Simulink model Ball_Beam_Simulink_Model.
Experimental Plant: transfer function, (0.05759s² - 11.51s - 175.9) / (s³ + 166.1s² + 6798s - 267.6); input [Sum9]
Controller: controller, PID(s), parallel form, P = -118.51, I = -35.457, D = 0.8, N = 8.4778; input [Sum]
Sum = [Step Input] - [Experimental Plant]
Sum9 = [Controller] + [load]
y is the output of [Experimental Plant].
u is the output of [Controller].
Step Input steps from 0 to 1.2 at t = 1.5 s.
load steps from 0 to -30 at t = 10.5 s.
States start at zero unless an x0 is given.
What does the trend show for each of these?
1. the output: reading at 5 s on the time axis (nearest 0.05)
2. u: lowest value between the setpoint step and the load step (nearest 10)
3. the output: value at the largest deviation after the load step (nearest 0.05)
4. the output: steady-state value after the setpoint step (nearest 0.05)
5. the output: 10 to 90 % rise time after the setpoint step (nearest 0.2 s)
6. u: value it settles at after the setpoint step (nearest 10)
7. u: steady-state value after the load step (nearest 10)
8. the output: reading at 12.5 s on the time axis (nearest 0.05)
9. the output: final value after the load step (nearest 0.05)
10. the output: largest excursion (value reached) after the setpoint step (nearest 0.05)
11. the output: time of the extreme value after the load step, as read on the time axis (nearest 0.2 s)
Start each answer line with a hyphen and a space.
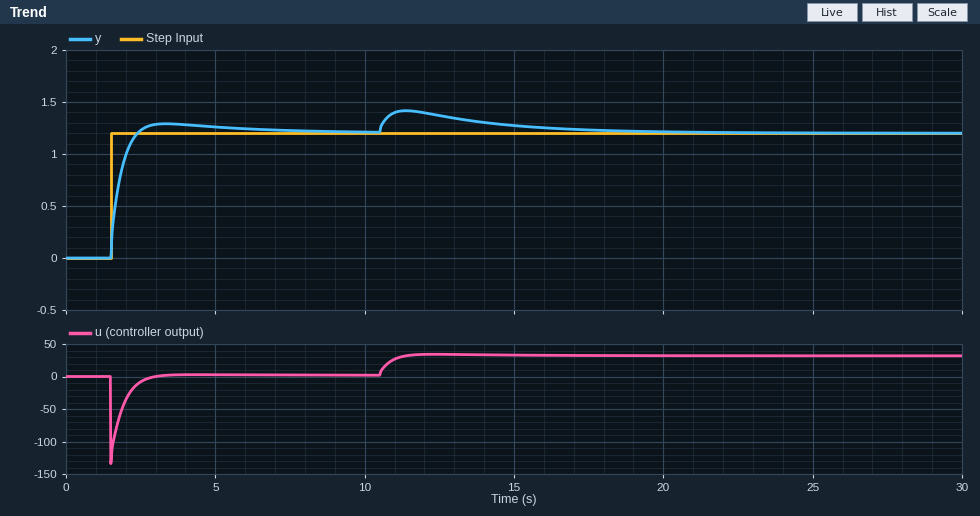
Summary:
- 1.25
- -130
- 1.40
- 1.20
- 0.6 s
- 0
- 30
- 1.35
- 1.20
- 1.30
- 11.4 s
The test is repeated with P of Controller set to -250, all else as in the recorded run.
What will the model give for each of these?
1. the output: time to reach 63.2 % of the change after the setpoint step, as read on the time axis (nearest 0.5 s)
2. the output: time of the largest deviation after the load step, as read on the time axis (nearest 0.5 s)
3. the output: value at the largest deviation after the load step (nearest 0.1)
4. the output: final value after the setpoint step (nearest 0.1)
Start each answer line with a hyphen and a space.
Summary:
- 1.5 s
- 11.0 s
- 1.3
- 1.2
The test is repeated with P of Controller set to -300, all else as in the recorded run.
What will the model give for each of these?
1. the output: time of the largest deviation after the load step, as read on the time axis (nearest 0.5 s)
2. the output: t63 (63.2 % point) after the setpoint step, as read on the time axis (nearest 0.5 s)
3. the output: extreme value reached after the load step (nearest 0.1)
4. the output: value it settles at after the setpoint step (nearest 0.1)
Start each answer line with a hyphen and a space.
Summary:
- 11.0 s
- 1.5 s
- 1.3
- 1.2
